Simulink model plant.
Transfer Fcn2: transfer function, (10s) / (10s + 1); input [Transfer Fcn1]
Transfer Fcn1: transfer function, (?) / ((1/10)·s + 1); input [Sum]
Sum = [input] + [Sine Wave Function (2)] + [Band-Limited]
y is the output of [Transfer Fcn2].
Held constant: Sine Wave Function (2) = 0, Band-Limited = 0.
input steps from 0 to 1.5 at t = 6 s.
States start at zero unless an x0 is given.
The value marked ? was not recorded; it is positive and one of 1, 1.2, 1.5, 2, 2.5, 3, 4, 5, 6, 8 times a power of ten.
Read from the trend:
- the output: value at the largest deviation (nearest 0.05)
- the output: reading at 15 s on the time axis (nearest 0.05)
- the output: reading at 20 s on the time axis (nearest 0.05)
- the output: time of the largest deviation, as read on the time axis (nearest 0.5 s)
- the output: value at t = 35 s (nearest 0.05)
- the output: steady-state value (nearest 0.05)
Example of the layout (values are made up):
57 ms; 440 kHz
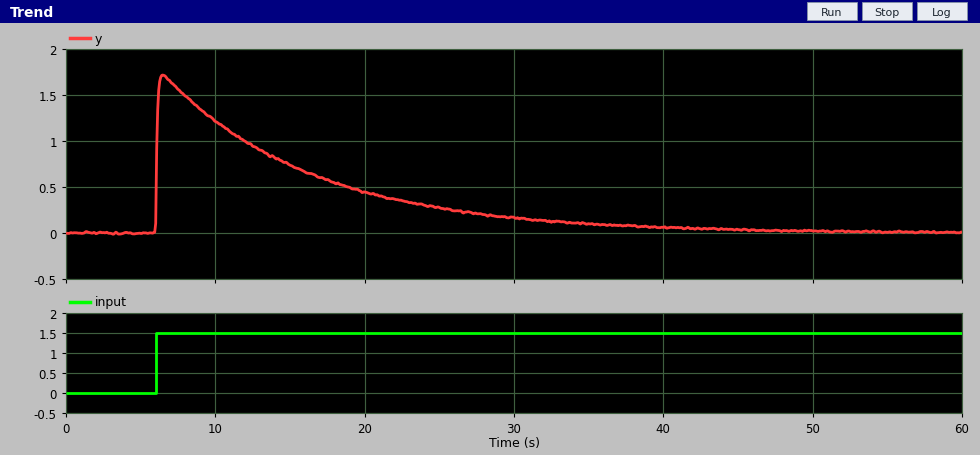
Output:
1.70; 0.75; 0.45; 6.5 s; 0.10; 0.00
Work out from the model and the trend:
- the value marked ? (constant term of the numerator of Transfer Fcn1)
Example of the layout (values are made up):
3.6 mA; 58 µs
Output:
1.2
